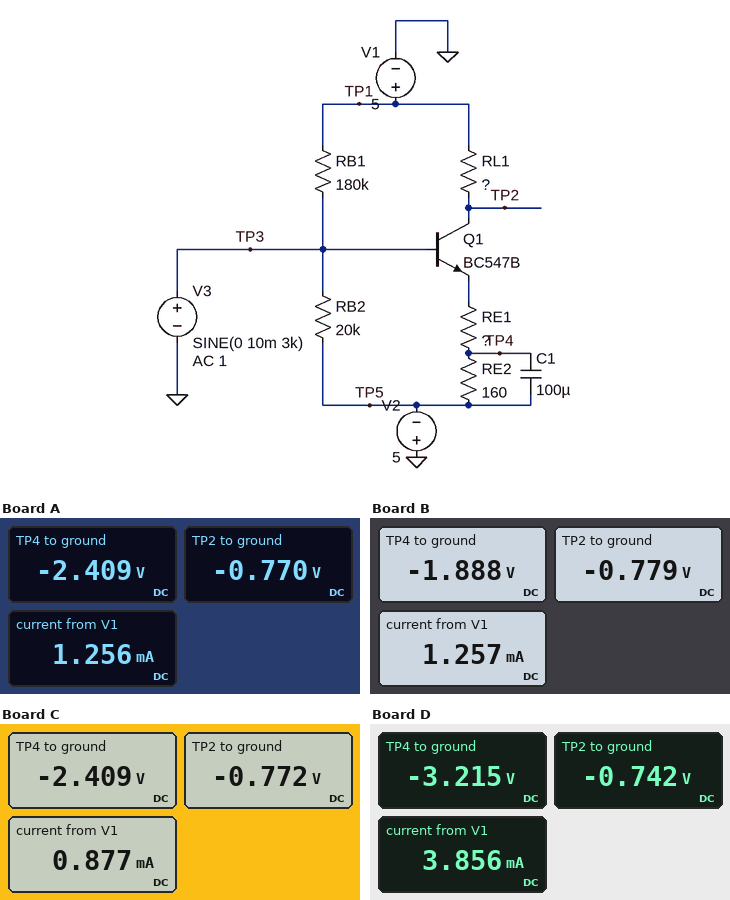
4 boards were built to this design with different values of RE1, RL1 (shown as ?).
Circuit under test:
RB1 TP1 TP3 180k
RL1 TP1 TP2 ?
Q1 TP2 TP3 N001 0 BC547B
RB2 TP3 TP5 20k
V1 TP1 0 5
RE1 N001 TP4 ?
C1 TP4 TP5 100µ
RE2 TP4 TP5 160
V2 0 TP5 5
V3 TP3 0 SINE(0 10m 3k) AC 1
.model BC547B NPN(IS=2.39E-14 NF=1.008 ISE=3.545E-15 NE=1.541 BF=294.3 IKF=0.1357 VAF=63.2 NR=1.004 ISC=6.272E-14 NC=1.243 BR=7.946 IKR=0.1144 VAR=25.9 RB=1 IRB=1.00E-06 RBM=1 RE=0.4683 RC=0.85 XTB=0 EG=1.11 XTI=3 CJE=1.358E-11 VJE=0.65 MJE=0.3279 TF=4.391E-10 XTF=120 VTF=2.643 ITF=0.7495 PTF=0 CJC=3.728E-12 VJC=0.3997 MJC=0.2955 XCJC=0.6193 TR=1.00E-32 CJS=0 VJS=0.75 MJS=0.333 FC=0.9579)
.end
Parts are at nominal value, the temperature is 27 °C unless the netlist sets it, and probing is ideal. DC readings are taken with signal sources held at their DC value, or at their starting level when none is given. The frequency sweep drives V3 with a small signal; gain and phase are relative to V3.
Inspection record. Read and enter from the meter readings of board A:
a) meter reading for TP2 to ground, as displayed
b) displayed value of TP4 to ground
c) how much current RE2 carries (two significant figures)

-0.770 V
-2.409 V
16 mA
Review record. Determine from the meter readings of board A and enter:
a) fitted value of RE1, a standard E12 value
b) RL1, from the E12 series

100 Ω
4.7 kΩ
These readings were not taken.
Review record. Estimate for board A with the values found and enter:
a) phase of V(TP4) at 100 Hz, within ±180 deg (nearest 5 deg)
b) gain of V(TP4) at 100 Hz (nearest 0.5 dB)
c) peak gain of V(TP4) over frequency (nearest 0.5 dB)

-75 deg
-16.5 dB
-4.5 dB
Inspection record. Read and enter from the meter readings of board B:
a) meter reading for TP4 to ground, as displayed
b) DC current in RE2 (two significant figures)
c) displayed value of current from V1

-1.888 V
19 mA
1.257 mA
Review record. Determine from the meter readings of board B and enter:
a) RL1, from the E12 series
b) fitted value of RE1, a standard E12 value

4.7 kΩ
56 Ω
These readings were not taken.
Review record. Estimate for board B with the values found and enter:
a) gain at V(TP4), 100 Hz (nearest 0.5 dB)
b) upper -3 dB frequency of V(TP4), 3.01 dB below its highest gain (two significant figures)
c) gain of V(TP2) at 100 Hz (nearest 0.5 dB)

-12.0 dB
37 Hz
-0.5 dB
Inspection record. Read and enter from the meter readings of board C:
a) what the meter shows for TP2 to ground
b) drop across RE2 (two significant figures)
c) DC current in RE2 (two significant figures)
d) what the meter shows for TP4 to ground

-0.772 V
2.6 V
16 mA
-2.409 V
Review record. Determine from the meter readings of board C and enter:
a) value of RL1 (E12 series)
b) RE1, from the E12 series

6.8 kΩ
100 Ω
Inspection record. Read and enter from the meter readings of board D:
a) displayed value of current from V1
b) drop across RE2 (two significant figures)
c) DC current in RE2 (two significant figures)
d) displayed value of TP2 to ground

3.856 mA
1.8 V
11 mA
-0.742 V
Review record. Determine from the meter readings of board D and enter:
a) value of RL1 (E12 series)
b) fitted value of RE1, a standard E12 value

1.5 kΩ
220 Ω
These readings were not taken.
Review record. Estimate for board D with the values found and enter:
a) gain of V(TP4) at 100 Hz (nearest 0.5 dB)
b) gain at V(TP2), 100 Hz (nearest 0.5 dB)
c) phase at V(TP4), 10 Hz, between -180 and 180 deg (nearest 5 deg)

-23.0 dB
0 dB
-30 deg
